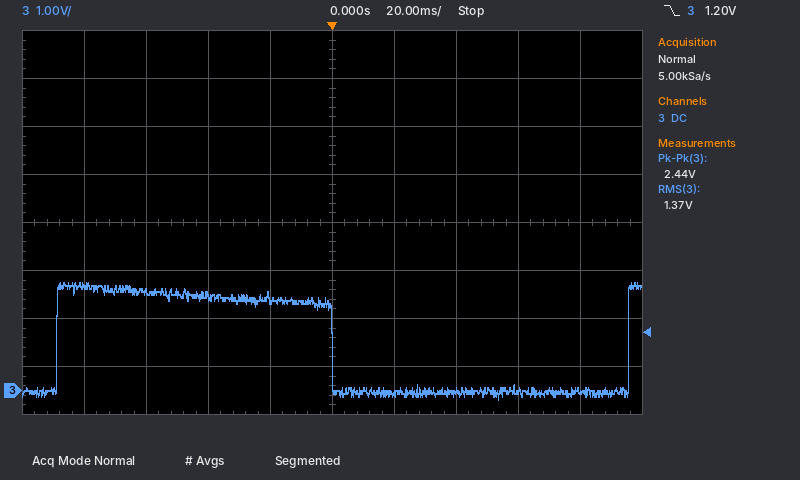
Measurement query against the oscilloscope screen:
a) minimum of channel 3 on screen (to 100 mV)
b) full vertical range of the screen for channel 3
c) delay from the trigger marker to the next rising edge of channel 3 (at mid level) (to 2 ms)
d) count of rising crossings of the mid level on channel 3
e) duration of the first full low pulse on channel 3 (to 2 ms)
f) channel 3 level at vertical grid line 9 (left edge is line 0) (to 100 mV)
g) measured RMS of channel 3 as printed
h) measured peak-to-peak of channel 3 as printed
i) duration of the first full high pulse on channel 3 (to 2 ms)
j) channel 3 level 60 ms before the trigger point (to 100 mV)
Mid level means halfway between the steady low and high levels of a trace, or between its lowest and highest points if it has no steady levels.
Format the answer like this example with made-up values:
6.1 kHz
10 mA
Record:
-200 mV
8 V
96 ms
2
96 ms
0.0 V
1.37 V
2.44 V
88 ms
2.1 V
